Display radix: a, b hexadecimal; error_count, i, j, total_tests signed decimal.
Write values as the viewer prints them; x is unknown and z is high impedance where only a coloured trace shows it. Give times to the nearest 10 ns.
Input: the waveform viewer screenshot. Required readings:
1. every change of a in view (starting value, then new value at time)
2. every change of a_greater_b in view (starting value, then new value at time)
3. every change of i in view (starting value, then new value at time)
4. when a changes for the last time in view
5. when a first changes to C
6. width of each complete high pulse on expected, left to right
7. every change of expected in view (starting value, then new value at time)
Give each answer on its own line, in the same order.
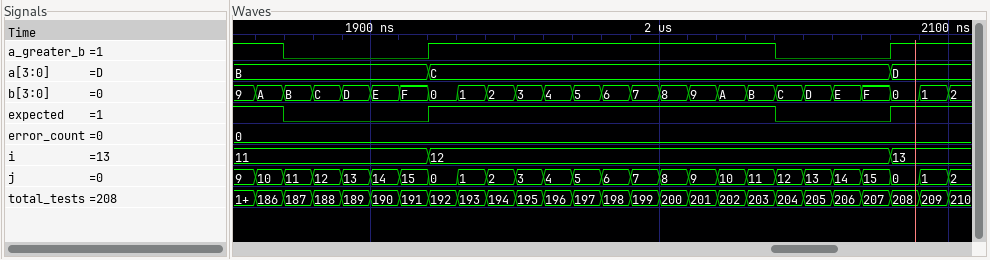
B, C at 1920 ns, D at 2080 ns
1, 0 at 1870 ns, 1 at 1920 ns, 0 at 2040 ns, 1 at 2080 ns
11, 12 at 1920 ns, 13 at 2080 ns
2080 ns
1920 ns
120 ns
1, 0 at 1870 ns, 1 at 1920 ns, 0 at 2040 ns, 1 at 2080 ns
